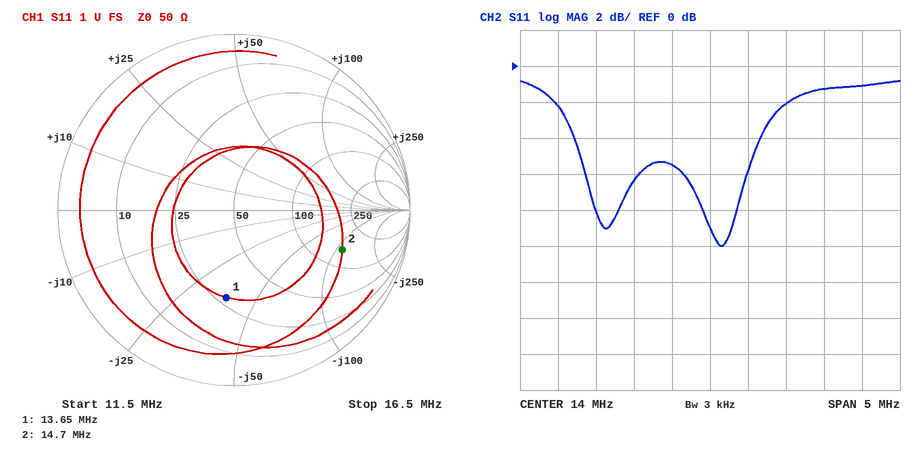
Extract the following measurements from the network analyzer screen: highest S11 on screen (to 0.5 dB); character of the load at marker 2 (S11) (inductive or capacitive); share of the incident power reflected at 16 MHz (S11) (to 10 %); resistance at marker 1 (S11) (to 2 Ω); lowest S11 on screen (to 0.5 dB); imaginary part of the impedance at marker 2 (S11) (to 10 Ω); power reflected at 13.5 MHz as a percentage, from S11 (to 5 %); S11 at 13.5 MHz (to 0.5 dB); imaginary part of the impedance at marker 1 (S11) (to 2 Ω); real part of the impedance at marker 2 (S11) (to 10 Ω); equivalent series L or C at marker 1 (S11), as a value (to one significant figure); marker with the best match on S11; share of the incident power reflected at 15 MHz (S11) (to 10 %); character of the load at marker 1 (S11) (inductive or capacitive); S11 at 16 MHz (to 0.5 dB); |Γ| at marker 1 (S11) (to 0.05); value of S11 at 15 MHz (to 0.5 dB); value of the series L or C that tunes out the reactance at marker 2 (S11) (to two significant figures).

-1.0 dB
capacitive
80 %
28 Ω
-10.0 dB
-110 Ω
30 %
-5.5 dB
-38 Ω
140 Ω
300 pF
marker 1
60 %
capacitive
-1.0 dB
0.50
-2.0 dB
1.2 µH
